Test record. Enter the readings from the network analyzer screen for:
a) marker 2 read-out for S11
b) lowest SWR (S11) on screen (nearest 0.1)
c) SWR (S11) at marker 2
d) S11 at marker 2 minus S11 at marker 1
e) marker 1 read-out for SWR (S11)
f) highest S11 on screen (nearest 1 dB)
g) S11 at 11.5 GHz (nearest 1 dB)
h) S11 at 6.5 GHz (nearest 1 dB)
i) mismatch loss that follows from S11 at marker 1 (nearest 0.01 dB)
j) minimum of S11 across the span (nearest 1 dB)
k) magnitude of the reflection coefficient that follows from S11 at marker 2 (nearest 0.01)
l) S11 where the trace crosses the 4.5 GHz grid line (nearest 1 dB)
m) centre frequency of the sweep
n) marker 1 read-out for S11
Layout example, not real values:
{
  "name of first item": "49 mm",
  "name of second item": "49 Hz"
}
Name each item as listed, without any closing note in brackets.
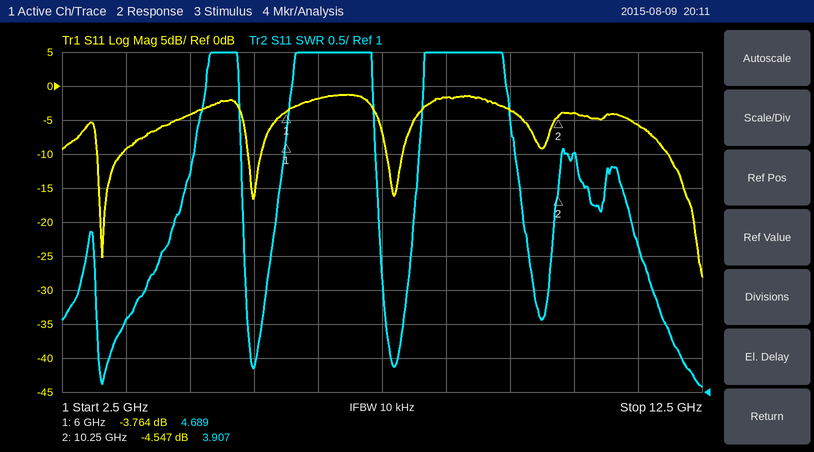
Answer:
{
  "marker 2 read-out for S11": "-4.547 dB",
  "lowest SWR (S11) on screen": "1.1",
  "SWR (S11) at marker 2": "3.907",
  "S11 at marker 2 minus S11 at marker 1": "-0.783 dB",
  "marker 1 read-out for SWR": "4.689",
  "highest S11 on screen": "-1 dB",
  "S11 at 11.5 GHz": "-6 dB",
  "S11 at 6.5 GHz": "-2 dB",
  "mismatch loss that follows from S11 at marker 1": "2.37 dB",
  "minimum of S11 across the span": "-28 dB",
  "magnitude of the reflection coefficient that follows from S11 at marker 2": "0.59",
  "S11 where the trace crosses the 4.5 GHz grid line": "-4 dB",
  "centre frequency of the sweep": "7.5 GHz",
  "marker 1 read-out for S11": "-3.764 dB"
}
